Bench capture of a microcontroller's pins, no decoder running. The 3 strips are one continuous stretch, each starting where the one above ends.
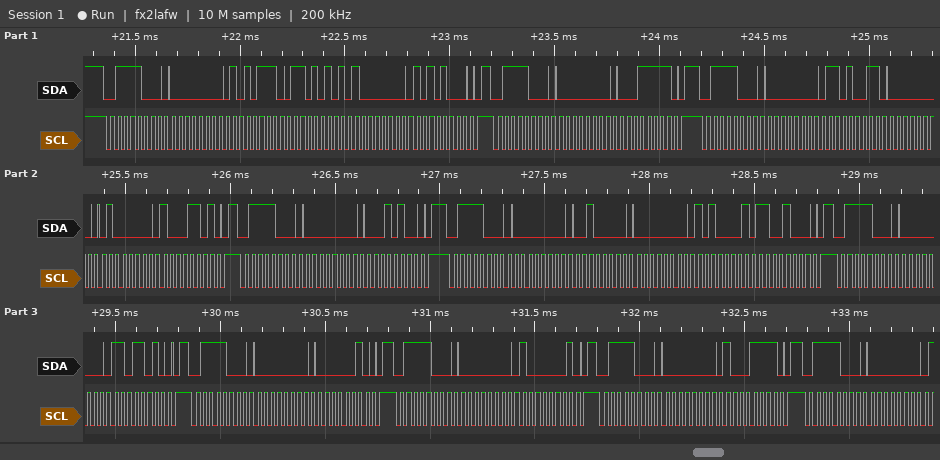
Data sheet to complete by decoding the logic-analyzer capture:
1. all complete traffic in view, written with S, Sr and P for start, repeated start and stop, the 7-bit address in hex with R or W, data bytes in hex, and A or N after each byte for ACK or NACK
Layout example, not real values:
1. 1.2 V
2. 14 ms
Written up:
1. S 3CW A 00 A AE A D5 A 80 A A8 A P S 3CW A 00 A 1F A P S 3CW A 00 A D3 A 00 A 40 A 8D A P S 3CW A 00 A 14 A P S 3CW A 00 A 20 A 00 A A1 A C8 A P S 3CW A 00 A DA A P S 3CW A 00 A 02 A P S 3CW A 00 A 81 A P S 3CW A 00 A 8F A P S 3CW A 00 A
